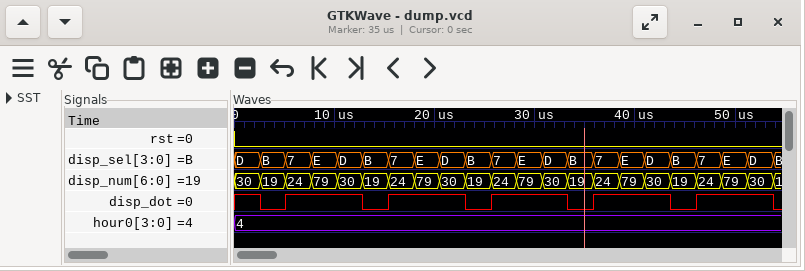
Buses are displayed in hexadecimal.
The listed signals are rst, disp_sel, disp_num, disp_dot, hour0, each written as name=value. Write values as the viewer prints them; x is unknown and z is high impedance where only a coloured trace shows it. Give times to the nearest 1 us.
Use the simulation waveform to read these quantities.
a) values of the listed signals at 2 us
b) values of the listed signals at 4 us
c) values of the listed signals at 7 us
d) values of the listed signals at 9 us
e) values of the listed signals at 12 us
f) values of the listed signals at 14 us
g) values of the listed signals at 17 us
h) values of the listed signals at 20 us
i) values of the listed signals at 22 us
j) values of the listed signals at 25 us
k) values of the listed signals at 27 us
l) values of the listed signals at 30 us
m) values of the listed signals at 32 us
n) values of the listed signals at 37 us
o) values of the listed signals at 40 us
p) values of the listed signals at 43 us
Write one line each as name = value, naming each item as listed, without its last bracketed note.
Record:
values of the listed signals at 2 us = rst=0, disp_sel=D, disp_num=30, disp_dot=1, hour0=4
values of the listed signals at 4 us = rst=0, disp_sel=B, disp_num=19, disp_dot=0, hour0=4
values of the listed signals at 7 us = rst=0, disp_sel=7, disp_num=24, disp_dot=1, hour0=4
values of the listed signals at 9 us = rst=0, disp_sel=E, disp_num=79, disp_dot=1, hour0=4
values of the listed signals at 12 us = rst=0, disp_sel=D, disp_num=30, disp_dot=1, hour0=4
values of the listed signals at 14 us = rst=0, disp_sel=B, disp_num=19, disp_dot=0, hour0=4
values of the listed signals at 17 us = rst=0, disp_sel=7, disp_num=24, disp_dot=1, hour0=4
values of the listed signals at 20 us = rst=0, disp_sel=E, disp_num=79, disp_dot=1, hour0=4
values of the listed signals at 22 us = rst=0, disp_sel=D, disp_num=30, disp_dot=1, hour0=4
values of the listed signals at 25 us = rst=0, disp_sel=B, disp_num=19, disp_dot=0, hour0=4
values of the listed signals at 27 us = rst=0, disp_sel=7, disp_num=24, disp_dot=1, hour0=4
values of the listed signals at 30 us = rst=0, disp_sel=E, disp_num=79, disp_dot=1, hour0=4
values of the listed signals at 32 us = rst=0, disp_sel=D, disp_num=30, disp_dot=1, hour0=4
values of the listed signals at 37 us = rst=0, disp_sel=7, disp_num=24, disp_dot=1, hour0=4
values of the listed signals at 40 us = rst=0, disp_sel=E, disp_num=79, disp_dot=1, hour0=4
values of the listed signals at 43 us = rst=0, disp_sel=D, disp_num=30, disp_dot=1, hour0=4
